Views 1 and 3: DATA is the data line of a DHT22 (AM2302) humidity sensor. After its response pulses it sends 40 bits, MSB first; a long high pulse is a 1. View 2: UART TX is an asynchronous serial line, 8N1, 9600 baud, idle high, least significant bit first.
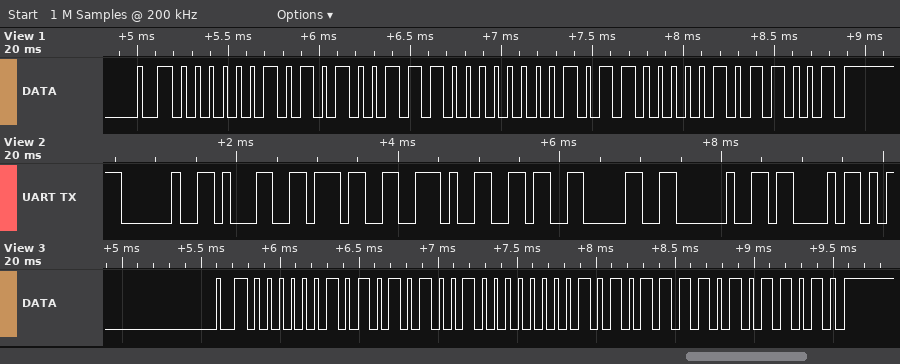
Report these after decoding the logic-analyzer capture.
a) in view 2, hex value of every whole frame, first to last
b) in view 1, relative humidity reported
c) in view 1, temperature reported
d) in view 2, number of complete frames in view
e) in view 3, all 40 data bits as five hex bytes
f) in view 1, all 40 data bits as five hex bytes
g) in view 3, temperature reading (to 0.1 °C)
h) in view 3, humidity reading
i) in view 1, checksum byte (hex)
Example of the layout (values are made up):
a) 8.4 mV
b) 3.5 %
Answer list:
a) 20 31 37 2E 36 30 20 43
b) 67.9 %
c) 17.6 °C
d) 8
e) 02 A9 00 AF 5A
f) 02 A7 00 B0 59
g) 17.5 °C
h) 68.1 %
i) 0x59
